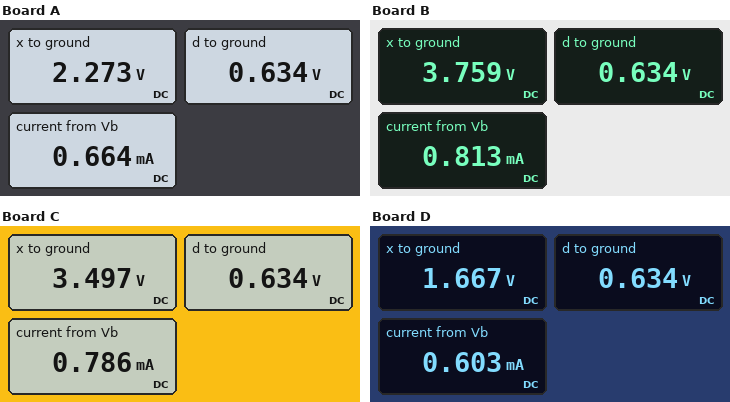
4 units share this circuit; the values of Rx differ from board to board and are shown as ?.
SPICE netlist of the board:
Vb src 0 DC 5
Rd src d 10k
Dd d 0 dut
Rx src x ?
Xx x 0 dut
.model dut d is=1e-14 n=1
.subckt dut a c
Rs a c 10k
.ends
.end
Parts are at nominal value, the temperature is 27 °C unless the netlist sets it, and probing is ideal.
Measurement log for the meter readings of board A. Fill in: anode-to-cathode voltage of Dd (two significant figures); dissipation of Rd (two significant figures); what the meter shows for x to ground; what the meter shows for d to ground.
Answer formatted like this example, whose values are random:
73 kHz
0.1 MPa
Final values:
630 mV
1.9 mW
2.273 V
0.634 V
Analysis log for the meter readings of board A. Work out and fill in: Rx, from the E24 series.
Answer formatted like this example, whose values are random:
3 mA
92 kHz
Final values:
12 kΩ
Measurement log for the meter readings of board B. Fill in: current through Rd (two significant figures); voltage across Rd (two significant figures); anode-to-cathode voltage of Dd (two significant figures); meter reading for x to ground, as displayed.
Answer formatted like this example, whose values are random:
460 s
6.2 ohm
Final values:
440 µA
4.4 V
630 mV
3.759 V
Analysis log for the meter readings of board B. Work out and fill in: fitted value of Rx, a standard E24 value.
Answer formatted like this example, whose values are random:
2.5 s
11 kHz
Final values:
3.3 kΩ
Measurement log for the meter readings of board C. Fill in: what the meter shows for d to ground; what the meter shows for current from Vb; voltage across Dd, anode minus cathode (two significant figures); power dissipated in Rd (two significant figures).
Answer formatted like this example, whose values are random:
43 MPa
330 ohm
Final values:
0.634 V
0.786 mA
630 mV
1.9 mW
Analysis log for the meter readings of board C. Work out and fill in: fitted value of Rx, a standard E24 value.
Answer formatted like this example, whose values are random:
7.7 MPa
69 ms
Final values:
4.3 kΩ
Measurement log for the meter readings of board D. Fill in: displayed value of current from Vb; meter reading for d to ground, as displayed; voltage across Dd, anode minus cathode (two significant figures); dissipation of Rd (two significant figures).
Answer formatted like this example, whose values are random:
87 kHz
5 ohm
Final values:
0.603 mA
0.634 V
630 mV
1.9 mW
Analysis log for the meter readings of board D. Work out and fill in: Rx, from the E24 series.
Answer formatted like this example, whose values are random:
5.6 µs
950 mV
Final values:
20 kΩ
